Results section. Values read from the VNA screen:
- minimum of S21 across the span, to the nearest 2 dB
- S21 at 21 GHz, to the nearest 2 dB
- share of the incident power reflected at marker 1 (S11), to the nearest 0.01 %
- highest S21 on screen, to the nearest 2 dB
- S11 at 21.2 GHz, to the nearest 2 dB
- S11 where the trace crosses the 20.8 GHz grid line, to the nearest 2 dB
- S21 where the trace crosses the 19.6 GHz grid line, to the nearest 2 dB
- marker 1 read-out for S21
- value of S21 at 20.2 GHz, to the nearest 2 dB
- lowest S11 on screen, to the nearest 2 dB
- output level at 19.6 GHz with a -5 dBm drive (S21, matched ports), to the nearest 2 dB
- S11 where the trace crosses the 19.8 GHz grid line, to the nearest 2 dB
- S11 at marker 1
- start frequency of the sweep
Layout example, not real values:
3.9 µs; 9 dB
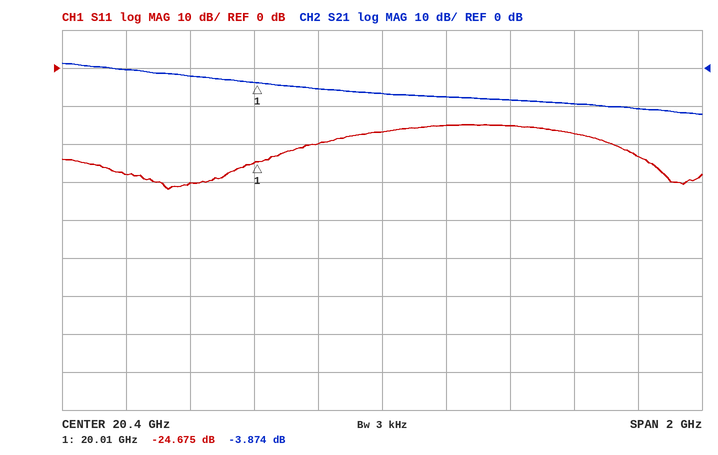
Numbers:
-12 dB; -10 dB; 0.34 %; 2 dB; -24 dB; -16 dB; 0 dB; -3.874 dB; -6 dB; -32 dB; -6 dBm; -30 dB; -24.675 dB; 19.4 GHz
